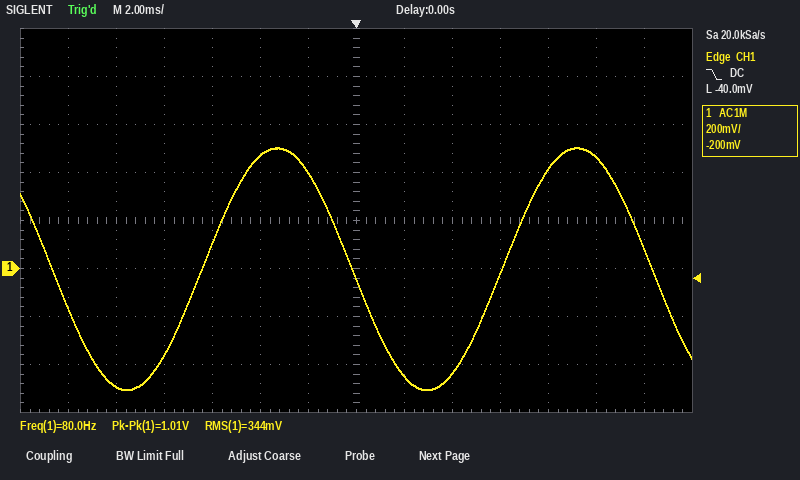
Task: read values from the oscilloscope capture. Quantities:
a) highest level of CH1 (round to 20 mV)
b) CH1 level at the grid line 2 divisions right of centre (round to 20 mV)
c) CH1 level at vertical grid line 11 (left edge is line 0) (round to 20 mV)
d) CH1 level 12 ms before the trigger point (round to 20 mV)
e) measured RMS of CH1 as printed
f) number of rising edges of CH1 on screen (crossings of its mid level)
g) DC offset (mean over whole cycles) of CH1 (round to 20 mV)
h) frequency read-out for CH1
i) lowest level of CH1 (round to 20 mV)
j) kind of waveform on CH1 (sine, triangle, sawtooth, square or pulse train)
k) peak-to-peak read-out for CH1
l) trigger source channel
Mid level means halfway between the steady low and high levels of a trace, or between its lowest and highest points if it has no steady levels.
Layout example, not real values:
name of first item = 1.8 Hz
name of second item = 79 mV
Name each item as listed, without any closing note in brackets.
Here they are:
highest level of CH1 = 500 mV
CH1 level at the grid line 2 divisions right of centre = -440 mV
CH1 level at vertical grid line 11 (left edge is line 0) = 420 mV
CH1 level 12 ms before the trigger point = -160 mV
measured RMS of CH1 as printed = 344 mV
number of rising edges of CH1 on screen = 2
DC offset (mean over whole cycles) of CH1 = 0 mV
frequency read-out for CH1 = 80.0 Hz
lowest level of CH1 = -500 mV
kind of waveform on CH1 = sine
peak-to-peak read-out for CH1 = 1.01 V
trigger source channel = CH1
